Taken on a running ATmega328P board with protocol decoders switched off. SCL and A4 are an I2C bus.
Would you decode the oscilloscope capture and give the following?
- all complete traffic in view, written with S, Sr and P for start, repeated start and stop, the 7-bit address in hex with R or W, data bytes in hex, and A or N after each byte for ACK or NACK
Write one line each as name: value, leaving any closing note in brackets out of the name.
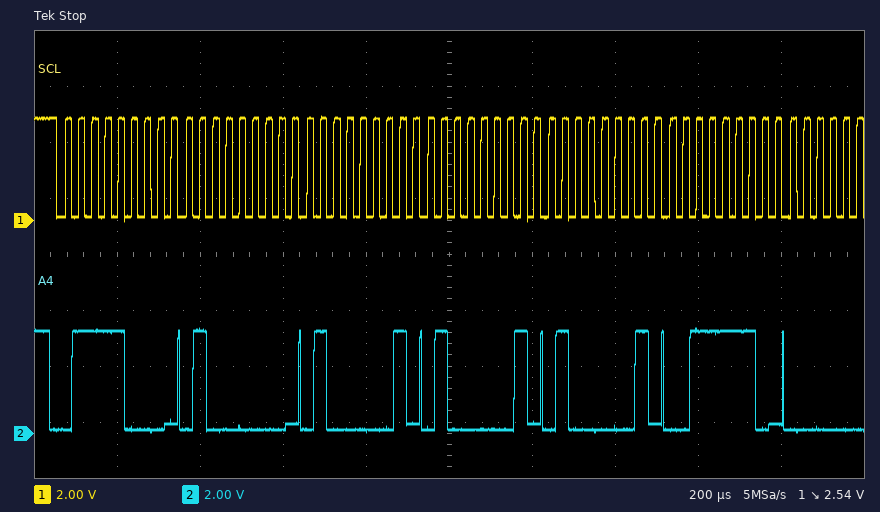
all complete traffic in view, written with S, Sr and P for start, repeated start and stop, the 7-bit address in hex with R or W, data bytes in hex, and A or N after each byte for ACK or NACK: S 3CW A 40 A 41 A 41 A 41 A 3E A
